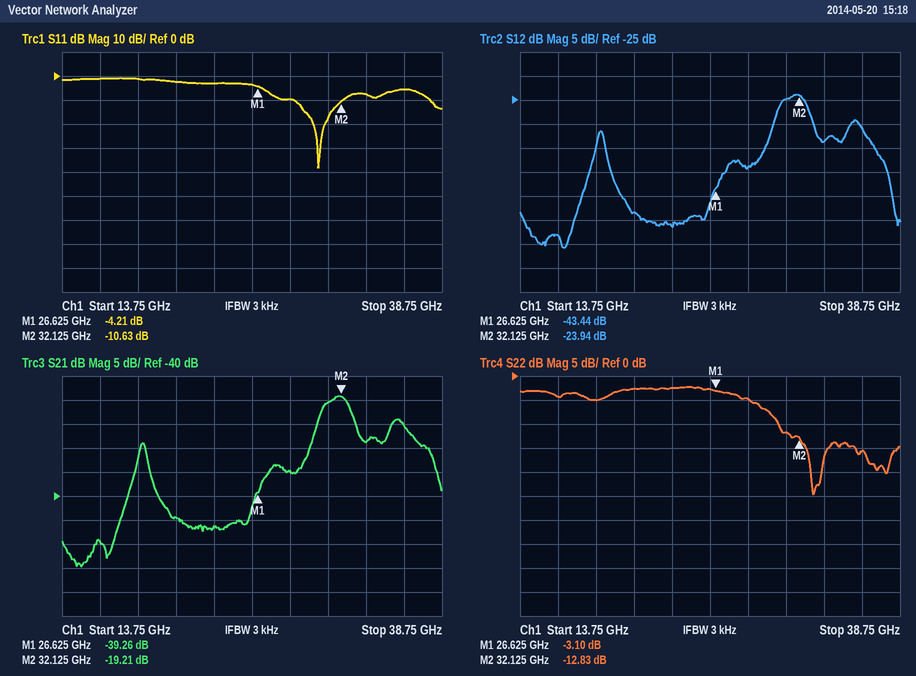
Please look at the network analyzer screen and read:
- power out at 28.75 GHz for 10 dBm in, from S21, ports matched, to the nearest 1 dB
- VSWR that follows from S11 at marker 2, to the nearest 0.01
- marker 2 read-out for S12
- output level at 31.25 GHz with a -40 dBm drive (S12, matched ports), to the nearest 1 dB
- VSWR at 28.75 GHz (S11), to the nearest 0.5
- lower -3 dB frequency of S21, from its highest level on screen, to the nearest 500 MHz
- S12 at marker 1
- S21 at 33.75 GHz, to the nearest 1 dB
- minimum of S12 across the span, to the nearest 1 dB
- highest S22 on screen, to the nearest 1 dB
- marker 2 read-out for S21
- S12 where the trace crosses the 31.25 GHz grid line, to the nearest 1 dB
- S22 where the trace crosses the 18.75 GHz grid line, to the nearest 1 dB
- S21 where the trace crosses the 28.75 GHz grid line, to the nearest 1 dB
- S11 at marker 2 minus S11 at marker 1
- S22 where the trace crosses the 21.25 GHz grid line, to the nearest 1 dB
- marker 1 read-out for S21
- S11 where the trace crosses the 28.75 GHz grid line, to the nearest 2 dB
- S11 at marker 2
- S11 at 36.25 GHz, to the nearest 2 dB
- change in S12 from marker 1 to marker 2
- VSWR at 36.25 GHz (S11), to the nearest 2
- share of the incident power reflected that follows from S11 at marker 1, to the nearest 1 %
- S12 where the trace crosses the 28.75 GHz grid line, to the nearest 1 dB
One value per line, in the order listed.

-25 dBm
1.83
-23.94 dB
-65 dBm
2.0
31.0 GHz
-43.44 dB
-29 dB
-56 dB
-2 dB
-19.21 dB
-25 dB
-5 dB
-35 dB
-6.42 dB
-3 dB
-39.26 dB
-10 dB
-10.63 dB
-6 dB
19.50 dB
4
38 %
-39 dB
